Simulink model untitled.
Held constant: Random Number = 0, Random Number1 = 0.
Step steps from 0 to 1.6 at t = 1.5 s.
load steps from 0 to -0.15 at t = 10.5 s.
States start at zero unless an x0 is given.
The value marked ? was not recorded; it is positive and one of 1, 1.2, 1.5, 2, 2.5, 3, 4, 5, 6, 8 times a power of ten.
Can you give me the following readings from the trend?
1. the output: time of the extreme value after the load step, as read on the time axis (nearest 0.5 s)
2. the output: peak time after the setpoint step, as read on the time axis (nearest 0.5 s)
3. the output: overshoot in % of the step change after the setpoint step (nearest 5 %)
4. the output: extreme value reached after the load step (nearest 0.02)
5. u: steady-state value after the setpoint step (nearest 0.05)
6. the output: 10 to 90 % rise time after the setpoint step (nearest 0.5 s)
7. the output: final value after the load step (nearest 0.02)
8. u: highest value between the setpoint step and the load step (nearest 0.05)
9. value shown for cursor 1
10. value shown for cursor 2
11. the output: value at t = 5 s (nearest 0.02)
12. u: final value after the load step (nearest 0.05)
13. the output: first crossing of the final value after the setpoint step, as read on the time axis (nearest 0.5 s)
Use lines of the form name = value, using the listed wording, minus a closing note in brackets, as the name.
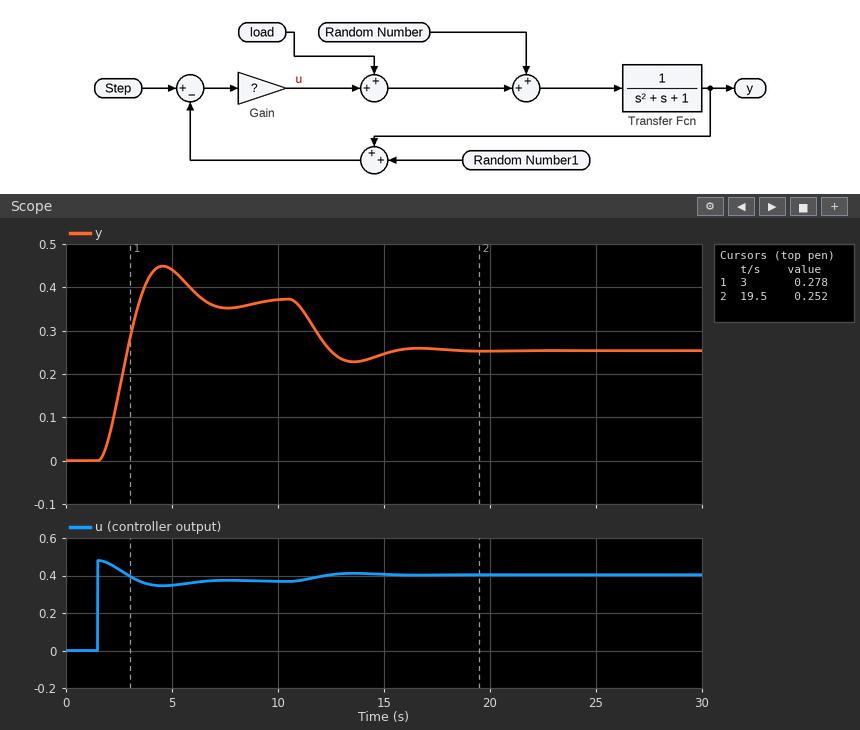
the output: time of the extreme value after the load step, as read on the time axis = 13.5 s
the output: peak time after the setpoint step, as read on the time axis = 4.5 s
the output: overshoot in % of the step change after the setpoint step = 20 %
the output: extreme value reached after the load step = 0.22
u: steady-state value after the setpoint step = 0.35
the output: 10 to 90 % rise time after the setpoint step = 1.5 s
the output: final value after the load step = 0.26
u: highest value between the setpoint step and the load step = 0.50
value shown for cursor 1 = 0.278
value shown for cursor 2 = 0.252
the output: value at t = 5 s = 0.44
u: final value after the load step = 0.40
the output: first crossing of the final value after the setpoint step, as read on the time axis = 3.5 s
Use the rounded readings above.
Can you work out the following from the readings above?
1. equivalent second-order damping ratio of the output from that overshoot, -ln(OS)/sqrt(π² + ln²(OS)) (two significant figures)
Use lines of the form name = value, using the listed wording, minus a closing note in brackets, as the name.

equivalent second-order damping ratio of the output from that overshoot, -ln(OS)/sqrt(π² + ln²(OS)) = 0.46
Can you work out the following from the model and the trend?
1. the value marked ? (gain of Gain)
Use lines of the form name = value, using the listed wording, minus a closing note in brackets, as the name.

the value marked ? = 0.3
